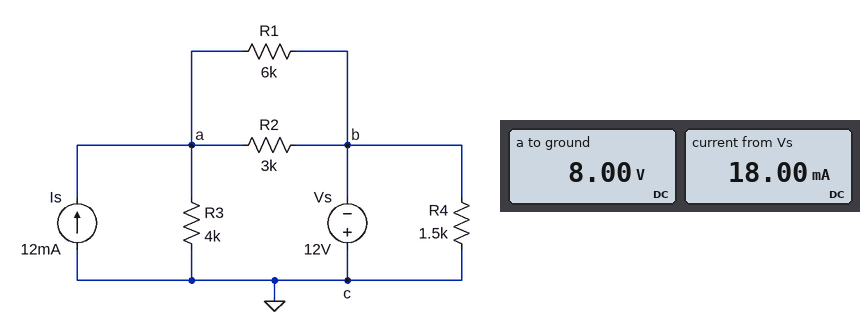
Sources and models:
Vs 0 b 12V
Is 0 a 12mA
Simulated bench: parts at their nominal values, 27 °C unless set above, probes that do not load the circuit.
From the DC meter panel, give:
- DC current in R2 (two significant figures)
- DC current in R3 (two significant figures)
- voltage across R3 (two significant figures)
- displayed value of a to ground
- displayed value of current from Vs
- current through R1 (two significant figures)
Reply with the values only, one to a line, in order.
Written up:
6.7 mA
2.0 mA
8.0 V
8.00 V
18.00 mA
3.3 mA
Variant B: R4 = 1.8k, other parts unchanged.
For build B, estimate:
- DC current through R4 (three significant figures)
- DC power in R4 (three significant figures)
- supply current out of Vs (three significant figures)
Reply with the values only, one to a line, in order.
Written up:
6.67 mA
80.0 mW
16.7 mA
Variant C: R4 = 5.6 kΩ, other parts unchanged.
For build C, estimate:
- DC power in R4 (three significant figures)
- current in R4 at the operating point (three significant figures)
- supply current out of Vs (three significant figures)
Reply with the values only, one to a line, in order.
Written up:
25.7 mW
2.14 mA
12.1 mA
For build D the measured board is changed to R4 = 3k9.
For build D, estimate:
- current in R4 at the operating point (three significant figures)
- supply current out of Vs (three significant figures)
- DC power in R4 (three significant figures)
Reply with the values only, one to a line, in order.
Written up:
3.08 mA
13.1 mA
36.9 mW
